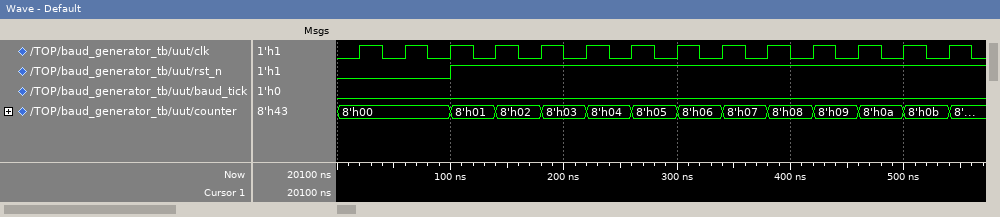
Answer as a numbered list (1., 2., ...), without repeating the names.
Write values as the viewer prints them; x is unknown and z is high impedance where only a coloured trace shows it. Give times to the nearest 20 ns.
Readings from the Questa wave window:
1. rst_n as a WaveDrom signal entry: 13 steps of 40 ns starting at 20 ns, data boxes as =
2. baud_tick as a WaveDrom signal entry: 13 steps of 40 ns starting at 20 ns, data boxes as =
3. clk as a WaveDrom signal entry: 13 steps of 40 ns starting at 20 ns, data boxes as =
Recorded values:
1. {name: 'rst_n', wave: '0.1..........'}
2. {name: 'baud_tick', wave: '0............'}
3. {name: 'clk', wave: 'p............'}
